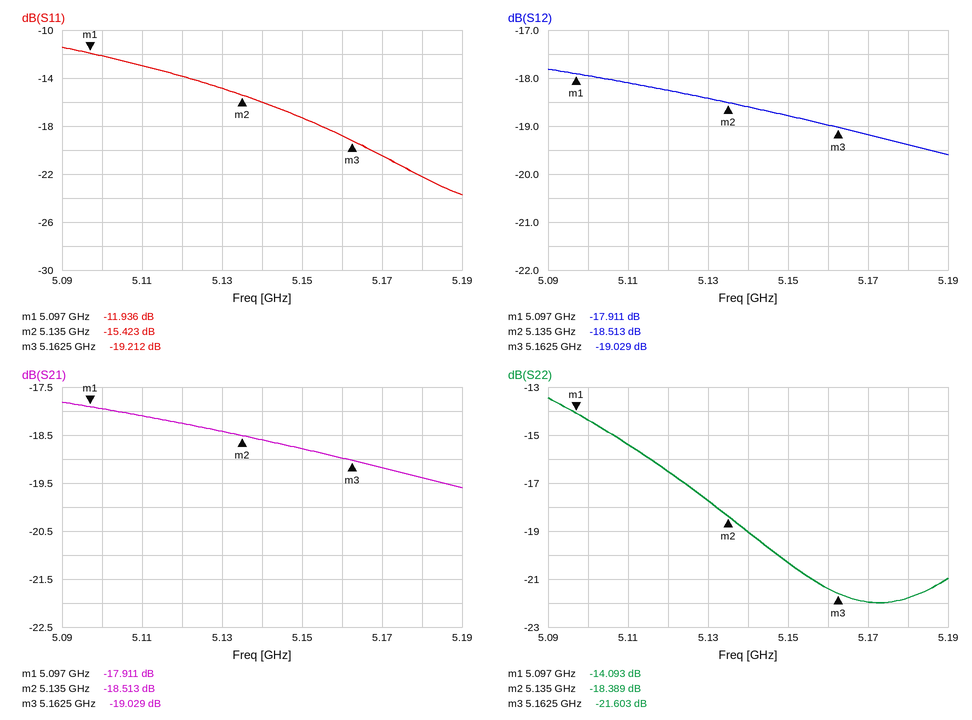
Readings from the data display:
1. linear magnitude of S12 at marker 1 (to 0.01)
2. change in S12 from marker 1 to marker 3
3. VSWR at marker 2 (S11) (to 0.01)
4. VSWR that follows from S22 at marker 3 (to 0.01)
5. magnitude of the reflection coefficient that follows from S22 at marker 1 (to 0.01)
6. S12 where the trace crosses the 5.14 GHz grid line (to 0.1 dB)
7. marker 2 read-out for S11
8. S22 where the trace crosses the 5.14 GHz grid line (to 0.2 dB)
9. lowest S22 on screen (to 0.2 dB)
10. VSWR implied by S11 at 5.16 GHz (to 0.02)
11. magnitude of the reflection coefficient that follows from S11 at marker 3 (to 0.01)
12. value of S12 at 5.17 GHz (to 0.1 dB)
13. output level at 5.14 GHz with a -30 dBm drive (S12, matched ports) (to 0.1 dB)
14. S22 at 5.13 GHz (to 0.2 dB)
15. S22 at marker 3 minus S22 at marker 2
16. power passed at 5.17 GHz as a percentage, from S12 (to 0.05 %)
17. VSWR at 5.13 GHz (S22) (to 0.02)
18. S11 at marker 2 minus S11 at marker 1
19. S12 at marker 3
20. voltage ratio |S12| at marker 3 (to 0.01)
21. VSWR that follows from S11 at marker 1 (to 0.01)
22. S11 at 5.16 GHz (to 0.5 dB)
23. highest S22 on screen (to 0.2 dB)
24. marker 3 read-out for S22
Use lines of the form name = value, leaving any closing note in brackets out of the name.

linear magnitude of S12 at marker 1 = 0.13
change in S12 from marker 1 to marker 3 = -1.118 dB
VSWR at marker 2 (S11) = 1.41
VSWR that follows from S22 at marker 3 = 1.18
magnitude of the reflection coefficient that follows from S22 at marker 1 = 0.20
S12 where the trace crosses the 5.14 GHz grid line = -18.6 dB
marker 2 read-out for S11 = -15.423 dB
S22 where the trace crosses the 5.14 GHz grid line = -19.0 dB
lowest S22 on screen = -22.0 dB
VSWR implied by S11 at 5.16 GHz = 1.26
magnitude of the reflection coefficient that follows from S11 at marker 3 = 0.11
value of S12 at 5.17 GHz = -19.2 dB
output level at 5.14 GHz with a -30 dBm drive (S12, matched ports) = -48.6 dBm
S22 at 5.13 GHz = -17.8 dB
S22 at marker 3 minus S22 at marker 2 = -3.214 dB
power passed at 5.17 GHz as a percentage, from S12 = 1.20 %
VSWR at 5.13 GHz (S22) = 1.30
S11 at marker 2 minus S11 at marker 1 = -3.487 dB
S12 at marker 3 = -19.029 dB
voltage ratio |S12| at marker 3 = 0.11
VSWR that follows from S11 at marker 1 = 1.68
S11 at 5.16 GHz = -19.0 dB
highest S22 on screen = -13.4 dB
marker 3 read-out for S22 = -21.603 dB
